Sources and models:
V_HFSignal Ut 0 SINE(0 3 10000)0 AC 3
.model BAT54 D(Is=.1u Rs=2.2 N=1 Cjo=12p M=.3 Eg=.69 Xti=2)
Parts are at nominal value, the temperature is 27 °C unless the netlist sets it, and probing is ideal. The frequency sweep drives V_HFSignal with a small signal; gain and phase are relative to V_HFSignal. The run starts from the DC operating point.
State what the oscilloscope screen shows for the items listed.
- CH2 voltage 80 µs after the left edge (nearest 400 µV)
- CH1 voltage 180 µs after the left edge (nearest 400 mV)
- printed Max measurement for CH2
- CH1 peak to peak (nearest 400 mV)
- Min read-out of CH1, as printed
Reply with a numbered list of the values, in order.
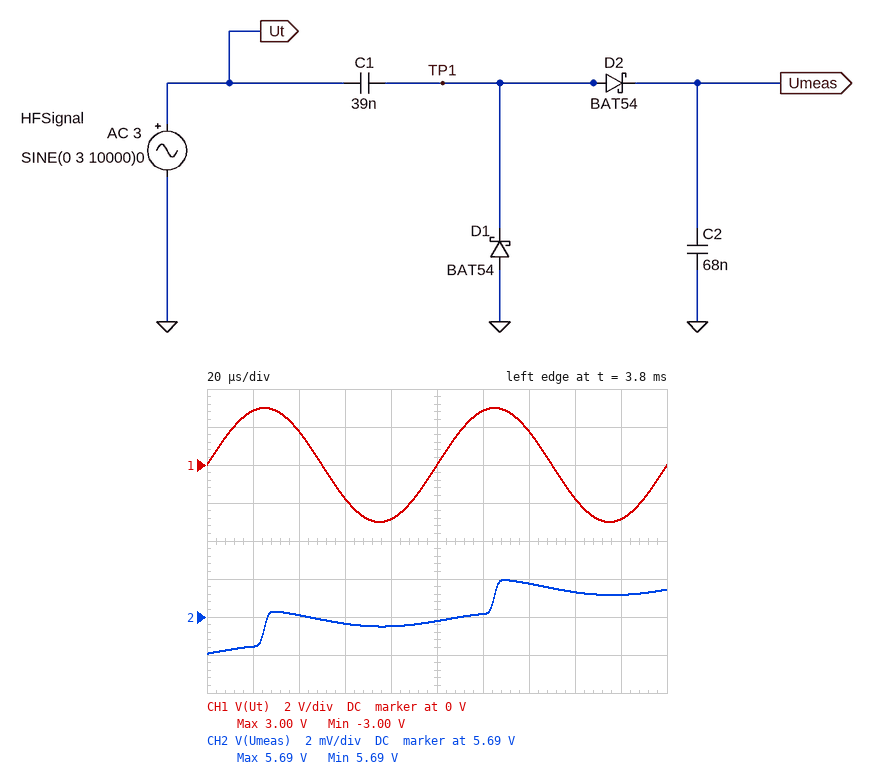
1. 5.6896 V
2. -2.8 V
3. 5.69 V
4. 6.0 V
5. -3.00 V
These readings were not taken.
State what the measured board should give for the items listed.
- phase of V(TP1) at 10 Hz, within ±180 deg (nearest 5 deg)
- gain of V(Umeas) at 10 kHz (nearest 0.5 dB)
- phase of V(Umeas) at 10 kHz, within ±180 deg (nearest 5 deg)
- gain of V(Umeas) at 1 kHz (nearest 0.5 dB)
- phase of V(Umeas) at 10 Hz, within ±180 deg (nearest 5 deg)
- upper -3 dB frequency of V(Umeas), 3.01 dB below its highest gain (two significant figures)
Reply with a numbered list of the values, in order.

1. 55 deg
2. -60.5 dB
3. -80 deg
4. -41.0 dB
5. 5 deg
6. 44 Hz
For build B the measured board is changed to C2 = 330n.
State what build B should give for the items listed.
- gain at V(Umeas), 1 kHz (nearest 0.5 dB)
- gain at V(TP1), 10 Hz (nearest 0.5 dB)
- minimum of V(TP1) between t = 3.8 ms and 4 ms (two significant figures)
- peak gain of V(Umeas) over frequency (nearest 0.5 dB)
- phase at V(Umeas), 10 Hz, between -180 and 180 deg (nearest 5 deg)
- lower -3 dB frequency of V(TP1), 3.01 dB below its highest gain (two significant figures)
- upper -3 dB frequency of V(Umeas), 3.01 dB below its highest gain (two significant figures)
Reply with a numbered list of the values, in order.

1. -54.5 dB
2. -10.5 dB
3. -230 mV
4. -25.0 dB
5. -10 deg
6. 32 Hz
7. 34 Hz
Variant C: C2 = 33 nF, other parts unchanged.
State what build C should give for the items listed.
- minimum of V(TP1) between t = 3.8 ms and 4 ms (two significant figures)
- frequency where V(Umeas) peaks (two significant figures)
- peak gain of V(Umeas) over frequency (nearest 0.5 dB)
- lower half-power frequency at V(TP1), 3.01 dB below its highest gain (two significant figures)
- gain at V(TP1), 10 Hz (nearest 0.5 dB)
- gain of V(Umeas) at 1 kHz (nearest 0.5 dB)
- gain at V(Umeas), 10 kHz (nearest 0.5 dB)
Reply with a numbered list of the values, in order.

1. -140 mV
2. 17 Hz
3. -8.5 dB
4. 36 Hz
5. -8.0 dB
6. -34.5 dB
7. -54.5 dB
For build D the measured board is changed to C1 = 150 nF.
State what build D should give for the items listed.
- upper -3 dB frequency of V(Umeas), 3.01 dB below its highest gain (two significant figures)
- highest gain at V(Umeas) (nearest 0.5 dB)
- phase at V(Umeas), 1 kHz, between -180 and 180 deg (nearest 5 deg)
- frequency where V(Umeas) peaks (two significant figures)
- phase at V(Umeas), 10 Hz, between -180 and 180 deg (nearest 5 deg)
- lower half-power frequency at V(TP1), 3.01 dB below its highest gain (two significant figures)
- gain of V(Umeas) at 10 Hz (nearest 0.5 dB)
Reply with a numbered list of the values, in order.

1. 19 Hz
2. -5.5 dB
3. -90 deg
4. 6.1 Hz
5. -20 deg
6. 8.8 Hz
7. -6.0 dB
